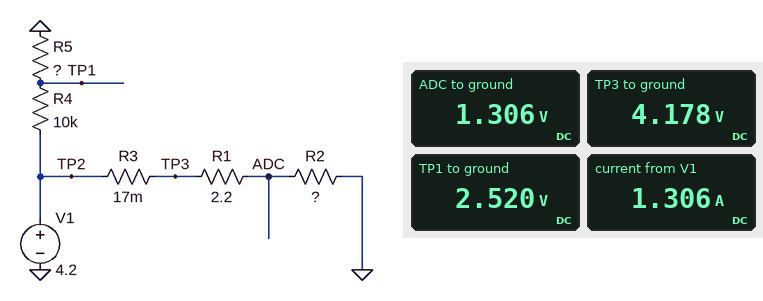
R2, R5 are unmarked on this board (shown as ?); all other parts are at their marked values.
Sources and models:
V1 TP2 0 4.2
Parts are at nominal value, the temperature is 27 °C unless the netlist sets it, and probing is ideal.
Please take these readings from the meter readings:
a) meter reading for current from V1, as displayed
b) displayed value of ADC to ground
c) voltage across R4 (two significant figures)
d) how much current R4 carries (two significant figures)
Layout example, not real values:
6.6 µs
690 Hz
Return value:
1.306 A
1.306 V
1.7 V
170 µA
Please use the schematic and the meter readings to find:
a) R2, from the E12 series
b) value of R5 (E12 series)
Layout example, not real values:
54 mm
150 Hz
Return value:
1 Ω
15 kΩ
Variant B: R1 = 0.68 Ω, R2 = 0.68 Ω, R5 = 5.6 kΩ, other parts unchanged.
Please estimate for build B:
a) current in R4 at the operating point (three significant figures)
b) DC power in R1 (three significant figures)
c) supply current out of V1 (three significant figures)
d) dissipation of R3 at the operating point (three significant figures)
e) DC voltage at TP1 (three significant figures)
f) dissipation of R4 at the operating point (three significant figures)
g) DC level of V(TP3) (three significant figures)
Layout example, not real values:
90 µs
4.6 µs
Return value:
269 µA
6.33 W
3.05 A
158 mW
1.51 V
725 µW
4.15 V
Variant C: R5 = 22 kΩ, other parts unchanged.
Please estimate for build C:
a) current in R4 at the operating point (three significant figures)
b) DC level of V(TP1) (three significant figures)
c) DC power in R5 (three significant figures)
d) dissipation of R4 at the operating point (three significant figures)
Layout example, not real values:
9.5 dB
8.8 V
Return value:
131 µA
2.89 V
379 µW
172 µW
